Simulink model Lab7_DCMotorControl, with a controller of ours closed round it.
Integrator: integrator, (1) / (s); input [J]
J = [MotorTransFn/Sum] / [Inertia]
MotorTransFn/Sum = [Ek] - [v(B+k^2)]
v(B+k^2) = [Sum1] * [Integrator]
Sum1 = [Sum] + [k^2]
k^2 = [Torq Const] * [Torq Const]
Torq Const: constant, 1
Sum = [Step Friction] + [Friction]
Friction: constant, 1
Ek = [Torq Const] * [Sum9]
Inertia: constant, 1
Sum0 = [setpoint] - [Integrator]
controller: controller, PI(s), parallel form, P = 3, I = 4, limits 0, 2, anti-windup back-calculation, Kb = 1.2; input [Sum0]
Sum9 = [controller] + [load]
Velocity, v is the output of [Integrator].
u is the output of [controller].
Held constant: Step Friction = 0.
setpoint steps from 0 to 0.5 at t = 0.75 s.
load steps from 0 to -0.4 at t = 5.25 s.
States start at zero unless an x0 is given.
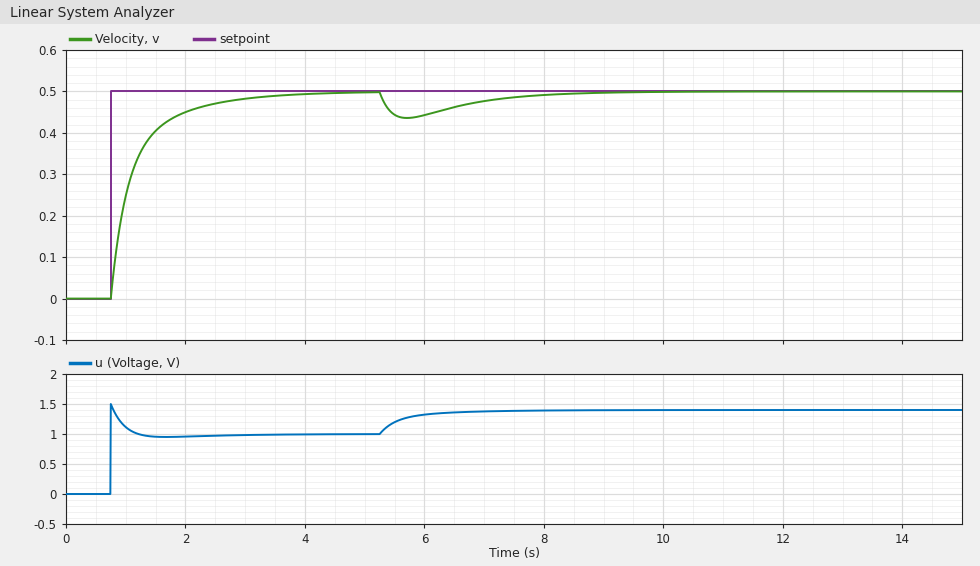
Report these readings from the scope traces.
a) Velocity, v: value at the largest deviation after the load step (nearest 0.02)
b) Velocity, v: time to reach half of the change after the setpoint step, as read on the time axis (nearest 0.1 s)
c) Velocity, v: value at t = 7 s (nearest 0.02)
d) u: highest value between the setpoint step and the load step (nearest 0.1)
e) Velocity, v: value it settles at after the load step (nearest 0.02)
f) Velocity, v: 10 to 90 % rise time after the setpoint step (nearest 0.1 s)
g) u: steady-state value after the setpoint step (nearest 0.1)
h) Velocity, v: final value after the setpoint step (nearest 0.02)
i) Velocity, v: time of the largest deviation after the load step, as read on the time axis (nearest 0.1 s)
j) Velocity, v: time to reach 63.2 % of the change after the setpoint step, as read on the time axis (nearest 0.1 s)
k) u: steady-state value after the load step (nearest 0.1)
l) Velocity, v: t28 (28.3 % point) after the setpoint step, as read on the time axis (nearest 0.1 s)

0.44
1.0 s
0.48
1.5
0.50
1.2 s
1.0
0.50
5.7 s
1.1 s
1.4
0.9 s
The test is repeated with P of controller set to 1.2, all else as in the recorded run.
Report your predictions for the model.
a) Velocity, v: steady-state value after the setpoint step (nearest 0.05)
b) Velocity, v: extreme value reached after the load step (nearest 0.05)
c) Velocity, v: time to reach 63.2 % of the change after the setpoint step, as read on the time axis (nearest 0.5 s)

0.50
0.40
1.5 s
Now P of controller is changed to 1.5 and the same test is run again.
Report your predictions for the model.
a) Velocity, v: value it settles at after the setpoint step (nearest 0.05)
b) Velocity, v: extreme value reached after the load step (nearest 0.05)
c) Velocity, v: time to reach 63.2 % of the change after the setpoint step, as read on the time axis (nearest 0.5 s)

0.50
0.40
1.5 s
